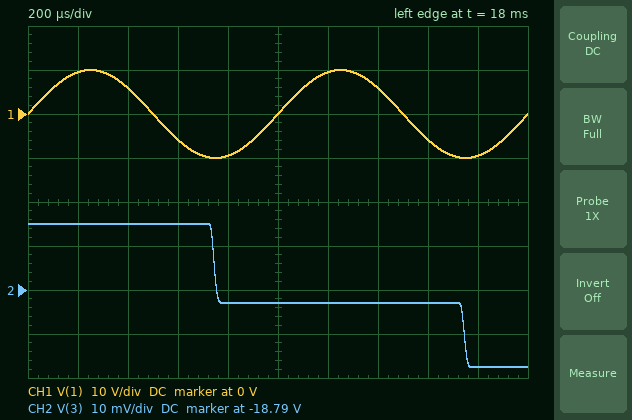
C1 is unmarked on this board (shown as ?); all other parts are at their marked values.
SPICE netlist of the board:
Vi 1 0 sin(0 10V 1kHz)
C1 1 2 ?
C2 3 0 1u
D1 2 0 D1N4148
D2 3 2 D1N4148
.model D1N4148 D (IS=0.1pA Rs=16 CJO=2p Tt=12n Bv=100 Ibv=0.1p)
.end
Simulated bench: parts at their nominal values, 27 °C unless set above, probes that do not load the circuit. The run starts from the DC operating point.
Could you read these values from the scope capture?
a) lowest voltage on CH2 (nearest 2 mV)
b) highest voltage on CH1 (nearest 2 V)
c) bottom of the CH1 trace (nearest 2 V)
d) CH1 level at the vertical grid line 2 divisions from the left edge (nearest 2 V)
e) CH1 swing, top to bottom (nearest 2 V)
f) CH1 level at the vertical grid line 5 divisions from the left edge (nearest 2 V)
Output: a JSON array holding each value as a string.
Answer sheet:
["-18.808 V", "10 V", "-10 V", "6 V", "20 V", "0 V"]
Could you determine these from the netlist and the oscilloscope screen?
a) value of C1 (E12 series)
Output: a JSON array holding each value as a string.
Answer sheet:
["390 nF"]
